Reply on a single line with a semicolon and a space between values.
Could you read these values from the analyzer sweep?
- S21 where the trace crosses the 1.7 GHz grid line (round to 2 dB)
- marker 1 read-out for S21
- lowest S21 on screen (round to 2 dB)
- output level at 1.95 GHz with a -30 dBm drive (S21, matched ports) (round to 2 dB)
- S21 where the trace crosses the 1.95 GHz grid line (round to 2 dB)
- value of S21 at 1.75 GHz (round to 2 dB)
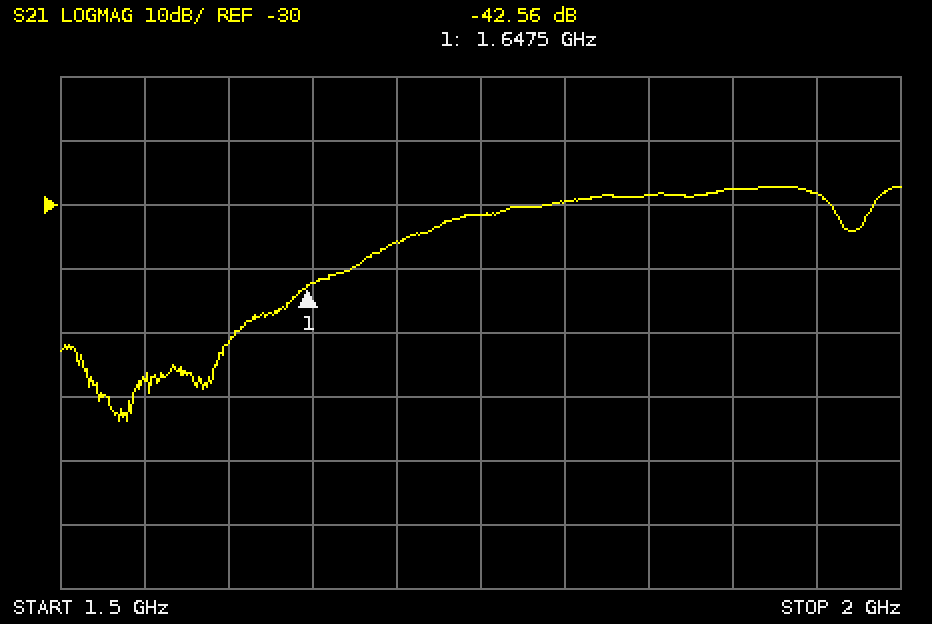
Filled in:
-36 dB; -42.56 dB; -64 dB; -58 dBm; -28 dB; -32 dB
